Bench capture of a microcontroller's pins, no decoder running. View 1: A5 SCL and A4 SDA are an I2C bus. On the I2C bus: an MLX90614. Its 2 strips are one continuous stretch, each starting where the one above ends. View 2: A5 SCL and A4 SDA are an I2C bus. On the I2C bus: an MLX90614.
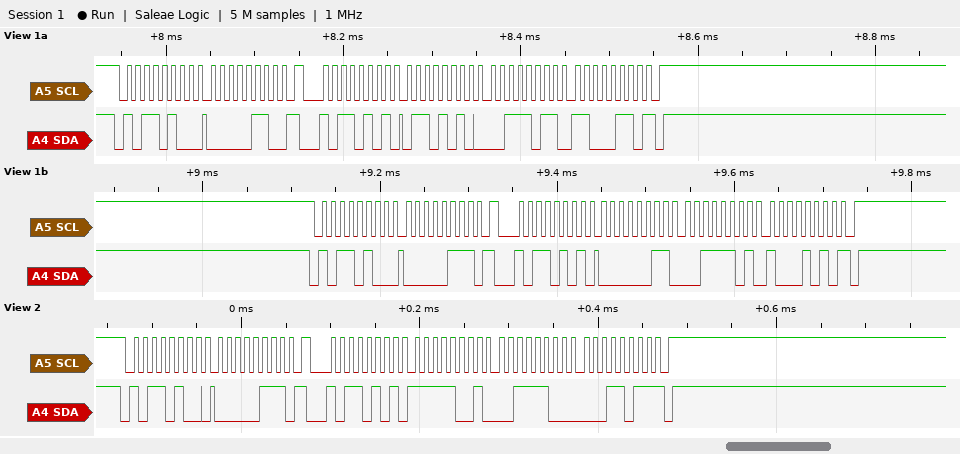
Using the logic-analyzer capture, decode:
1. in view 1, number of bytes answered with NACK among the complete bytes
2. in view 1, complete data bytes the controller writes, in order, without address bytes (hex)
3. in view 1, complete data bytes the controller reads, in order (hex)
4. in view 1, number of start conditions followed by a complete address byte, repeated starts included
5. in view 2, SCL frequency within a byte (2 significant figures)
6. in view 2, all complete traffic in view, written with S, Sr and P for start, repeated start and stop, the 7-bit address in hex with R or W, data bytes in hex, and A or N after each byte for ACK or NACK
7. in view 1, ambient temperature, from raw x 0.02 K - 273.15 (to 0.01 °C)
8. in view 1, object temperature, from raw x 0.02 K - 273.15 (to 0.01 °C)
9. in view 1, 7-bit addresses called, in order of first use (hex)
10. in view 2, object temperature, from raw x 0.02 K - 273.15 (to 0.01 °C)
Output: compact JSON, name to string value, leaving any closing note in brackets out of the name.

{"in view 1, number of bytes answered with NACK among the complete bytes": "2", "in view 1, complete data bytes the controller writes, in order, without address bytes": "06 07", "in view 1, complete data bytes the controller reads, in order": "6A 3B C6 03 3D 8A", "in view 1, number of start conditions followed by a complete address byte, repeated starts included": "4", "in view 2, SCL frequency within a byte": "100 kHz", "in view 2, all complete traffic in view, written with S, Sr and P for start, repeated start and stop, the 7-bit address in hex with R or W, data bytes in hex, and A or N after each byte for ACK or NACK": "S 5AW A 07 A Sr 5AR A F9 A 3C A 1B N P", "in view 1, ambient temperature, from raw x 0.02 K - 273.15": "31.05 °C", "in view 1, object temperature, from raw x 0.02 K - 273.15": "39.23 °C", "in view 1, 7-bit addresses called, in order of first use": "0x5A", "in view 2, object temperature, from raw x 0.02 K - 273.15": "39.03 °C"}
